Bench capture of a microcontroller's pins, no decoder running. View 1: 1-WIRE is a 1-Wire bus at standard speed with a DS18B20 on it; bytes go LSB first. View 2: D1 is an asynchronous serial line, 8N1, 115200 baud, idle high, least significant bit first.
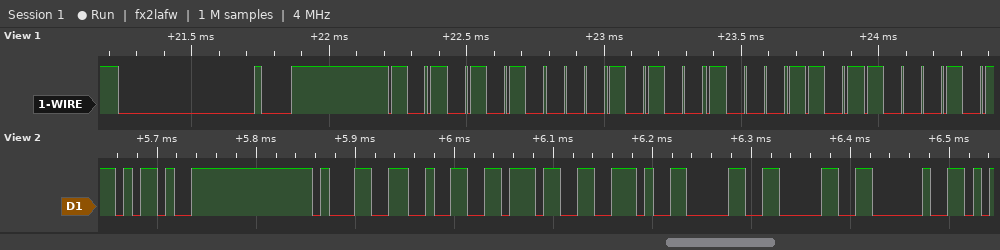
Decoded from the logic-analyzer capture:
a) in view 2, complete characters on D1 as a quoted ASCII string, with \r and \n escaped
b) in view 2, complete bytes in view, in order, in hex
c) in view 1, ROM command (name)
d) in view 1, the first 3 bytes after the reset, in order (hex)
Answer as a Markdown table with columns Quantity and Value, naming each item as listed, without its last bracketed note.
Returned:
| Quantity | Value |
|---|---|
| in view 2, complete characters on D1 as a quoted ASCII string, with \r and \n escaped | "-127.00 " |
| in view 2, complete bytes in view, in order, in hex | 2D 31 32 37 2E 30 30 20 |
| in view 1, ROM command | Match ROM |
| in view 1, the first 3 bytes after the reset, in order | 55 28 B1 |
